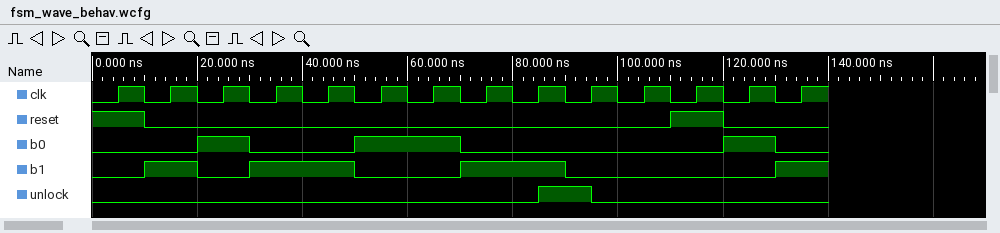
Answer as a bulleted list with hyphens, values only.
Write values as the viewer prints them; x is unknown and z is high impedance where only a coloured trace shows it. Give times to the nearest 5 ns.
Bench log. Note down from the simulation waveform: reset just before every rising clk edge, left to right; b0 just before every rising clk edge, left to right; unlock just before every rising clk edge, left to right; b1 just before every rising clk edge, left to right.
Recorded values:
- 1 0 0 0 0 0 0 0 0 0 0 1 0 0
- 0 0 1 0 0 1 1 0 0 0 0 0 1 0
- 0 0 0 0 0 0 0 0 0 1 0 0 0 0
- 0 1 0 1 1 0 0 1 1 0 0 0 0 1
